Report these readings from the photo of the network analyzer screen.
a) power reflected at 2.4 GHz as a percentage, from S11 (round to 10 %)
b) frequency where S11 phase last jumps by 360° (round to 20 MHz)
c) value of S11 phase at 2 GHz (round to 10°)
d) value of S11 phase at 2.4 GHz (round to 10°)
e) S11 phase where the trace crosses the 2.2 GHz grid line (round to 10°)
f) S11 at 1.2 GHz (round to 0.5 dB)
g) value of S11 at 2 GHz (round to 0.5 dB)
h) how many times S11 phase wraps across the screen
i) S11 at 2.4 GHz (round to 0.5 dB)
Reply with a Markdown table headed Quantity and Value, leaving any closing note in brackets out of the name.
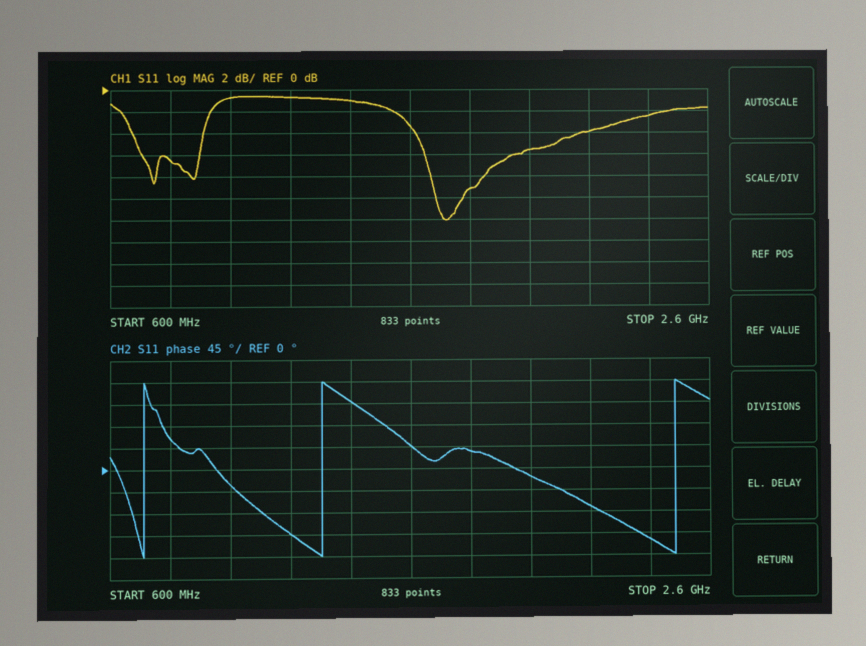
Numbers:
| Quantity | Value |
|---|---|
| power reflected at 2.4 GHz as a percentage, from S11 | 60 % |
| frequency where S11 phase last jumps by 360° | 2.48 GHz |
| value of S11 phase at 2 GHz | -20° |
| value of S11 phase at 2.4 GHz | -150° |
| S11 phase where the trace crosses the 2.2 GHz grid line | -80° |
| S11 at 1.2 GHz | -0.5 dB |
| value of S11 at 2 GHz | -5.5 dB |
| how many times S11 phase wraps across the screen | 3 |
| S11 at 2.4 GHz | -2.5 dB |
